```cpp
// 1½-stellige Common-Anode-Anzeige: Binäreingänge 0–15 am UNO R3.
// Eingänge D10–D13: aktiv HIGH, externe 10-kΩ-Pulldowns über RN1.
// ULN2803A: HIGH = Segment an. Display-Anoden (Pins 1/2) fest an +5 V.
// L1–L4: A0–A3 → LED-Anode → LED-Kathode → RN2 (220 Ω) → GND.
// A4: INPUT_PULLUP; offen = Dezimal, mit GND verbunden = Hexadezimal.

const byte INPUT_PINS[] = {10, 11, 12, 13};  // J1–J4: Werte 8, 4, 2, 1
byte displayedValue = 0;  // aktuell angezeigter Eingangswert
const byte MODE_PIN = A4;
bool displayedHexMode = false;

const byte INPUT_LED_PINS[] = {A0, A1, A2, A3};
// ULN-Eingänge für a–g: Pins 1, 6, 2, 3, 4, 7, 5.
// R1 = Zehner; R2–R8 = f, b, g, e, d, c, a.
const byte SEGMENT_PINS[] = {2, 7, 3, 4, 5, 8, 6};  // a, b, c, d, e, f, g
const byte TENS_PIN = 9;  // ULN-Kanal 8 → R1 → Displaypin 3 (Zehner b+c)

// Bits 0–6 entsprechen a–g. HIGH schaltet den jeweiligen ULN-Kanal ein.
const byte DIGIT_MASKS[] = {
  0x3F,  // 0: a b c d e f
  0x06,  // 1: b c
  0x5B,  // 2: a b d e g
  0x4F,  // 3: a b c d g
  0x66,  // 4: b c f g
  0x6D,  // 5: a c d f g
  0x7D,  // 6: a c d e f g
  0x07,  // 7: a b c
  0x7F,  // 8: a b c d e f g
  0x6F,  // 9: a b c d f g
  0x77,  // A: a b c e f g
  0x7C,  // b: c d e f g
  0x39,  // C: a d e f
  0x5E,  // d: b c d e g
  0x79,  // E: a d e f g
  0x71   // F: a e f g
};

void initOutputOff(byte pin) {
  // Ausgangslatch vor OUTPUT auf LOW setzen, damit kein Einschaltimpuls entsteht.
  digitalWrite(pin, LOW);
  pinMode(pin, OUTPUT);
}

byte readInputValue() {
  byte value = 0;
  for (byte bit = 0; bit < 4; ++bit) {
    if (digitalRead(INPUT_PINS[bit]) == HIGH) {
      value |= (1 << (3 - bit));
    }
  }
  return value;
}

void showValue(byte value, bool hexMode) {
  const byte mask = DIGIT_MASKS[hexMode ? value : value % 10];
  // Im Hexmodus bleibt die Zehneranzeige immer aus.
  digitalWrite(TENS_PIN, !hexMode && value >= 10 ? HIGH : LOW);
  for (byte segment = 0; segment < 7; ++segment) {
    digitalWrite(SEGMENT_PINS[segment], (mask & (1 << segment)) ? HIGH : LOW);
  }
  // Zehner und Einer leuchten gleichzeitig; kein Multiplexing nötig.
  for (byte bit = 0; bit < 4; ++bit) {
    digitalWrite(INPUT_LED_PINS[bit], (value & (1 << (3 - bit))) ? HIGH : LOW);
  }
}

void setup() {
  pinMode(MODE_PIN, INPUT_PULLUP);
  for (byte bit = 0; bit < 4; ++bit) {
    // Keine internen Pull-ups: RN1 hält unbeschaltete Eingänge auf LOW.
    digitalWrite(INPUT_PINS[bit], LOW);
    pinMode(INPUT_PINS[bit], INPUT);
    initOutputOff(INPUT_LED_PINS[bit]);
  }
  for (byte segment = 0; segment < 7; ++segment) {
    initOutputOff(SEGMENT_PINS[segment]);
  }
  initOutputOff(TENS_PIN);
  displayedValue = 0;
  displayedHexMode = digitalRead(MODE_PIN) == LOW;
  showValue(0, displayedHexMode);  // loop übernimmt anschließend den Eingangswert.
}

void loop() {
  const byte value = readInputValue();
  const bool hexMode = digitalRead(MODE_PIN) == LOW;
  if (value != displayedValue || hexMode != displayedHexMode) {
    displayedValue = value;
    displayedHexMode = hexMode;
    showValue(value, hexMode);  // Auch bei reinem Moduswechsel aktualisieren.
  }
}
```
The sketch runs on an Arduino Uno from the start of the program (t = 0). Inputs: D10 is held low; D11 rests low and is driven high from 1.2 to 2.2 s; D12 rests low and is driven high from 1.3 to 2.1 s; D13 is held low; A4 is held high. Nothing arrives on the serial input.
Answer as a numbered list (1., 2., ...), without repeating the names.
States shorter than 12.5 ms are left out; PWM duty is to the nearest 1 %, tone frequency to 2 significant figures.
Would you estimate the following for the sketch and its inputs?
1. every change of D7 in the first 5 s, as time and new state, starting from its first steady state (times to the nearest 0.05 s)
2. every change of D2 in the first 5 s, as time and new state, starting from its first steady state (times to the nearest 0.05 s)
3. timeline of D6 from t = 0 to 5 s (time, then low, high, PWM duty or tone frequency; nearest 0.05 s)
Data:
1. 0 s high; 1.3 s low; 2.1 s high
2. 0 s high; 1.2 s low; 1.3 s high; 2.1 s low; 2.2 s high
3. 0 s low; 1.2 s high; 2.2 s low
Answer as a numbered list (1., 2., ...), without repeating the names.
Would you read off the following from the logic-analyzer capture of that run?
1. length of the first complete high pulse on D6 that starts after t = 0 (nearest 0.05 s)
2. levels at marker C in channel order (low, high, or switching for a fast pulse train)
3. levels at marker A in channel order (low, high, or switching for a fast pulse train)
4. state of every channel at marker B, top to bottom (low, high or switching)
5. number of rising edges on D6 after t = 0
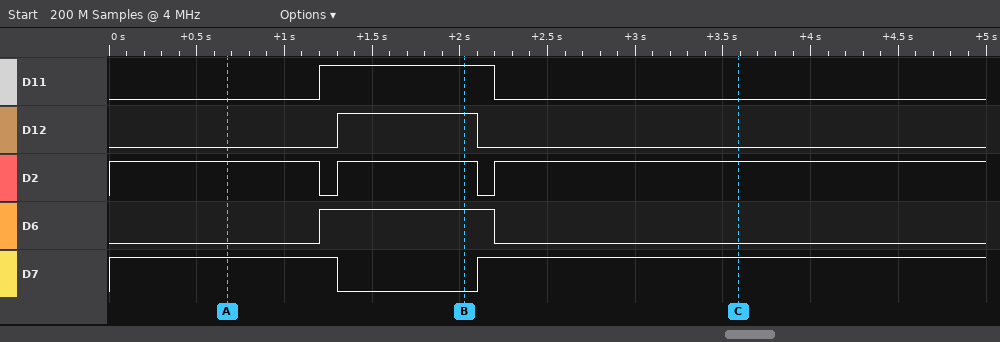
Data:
1. 1.00 s
2. D11 low, D12 low, D2 high, D6 low, D7 high
3. D11 low, D12 low, D2 high, D6 low, D7 high
4. D11 high, D12 high, D2 high, D6 high, D7 low
5. 1
